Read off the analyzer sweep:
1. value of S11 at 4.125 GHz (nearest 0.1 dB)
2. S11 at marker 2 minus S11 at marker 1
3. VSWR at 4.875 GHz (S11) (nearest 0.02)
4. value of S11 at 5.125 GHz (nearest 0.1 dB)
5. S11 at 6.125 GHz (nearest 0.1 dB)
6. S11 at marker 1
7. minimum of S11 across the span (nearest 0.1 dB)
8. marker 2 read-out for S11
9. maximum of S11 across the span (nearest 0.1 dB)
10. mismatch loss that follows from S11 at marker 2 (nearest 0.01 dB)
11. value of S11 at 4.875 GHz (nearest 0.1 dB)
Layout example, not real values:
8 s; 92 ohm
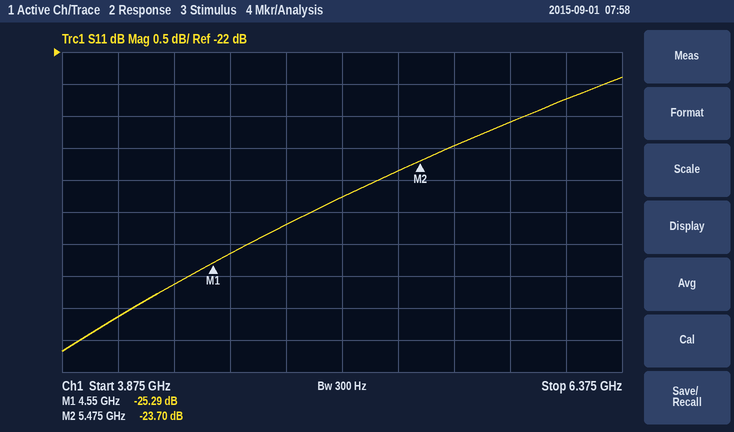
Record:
-26.1 dB; 1.59 dB; 1.12; -24.3 dB; -22.7 dB; -25.29 dB; -26.7 dB; -23.70 dB; -22.4 dB; 0.02 dB; -24.7 dB
